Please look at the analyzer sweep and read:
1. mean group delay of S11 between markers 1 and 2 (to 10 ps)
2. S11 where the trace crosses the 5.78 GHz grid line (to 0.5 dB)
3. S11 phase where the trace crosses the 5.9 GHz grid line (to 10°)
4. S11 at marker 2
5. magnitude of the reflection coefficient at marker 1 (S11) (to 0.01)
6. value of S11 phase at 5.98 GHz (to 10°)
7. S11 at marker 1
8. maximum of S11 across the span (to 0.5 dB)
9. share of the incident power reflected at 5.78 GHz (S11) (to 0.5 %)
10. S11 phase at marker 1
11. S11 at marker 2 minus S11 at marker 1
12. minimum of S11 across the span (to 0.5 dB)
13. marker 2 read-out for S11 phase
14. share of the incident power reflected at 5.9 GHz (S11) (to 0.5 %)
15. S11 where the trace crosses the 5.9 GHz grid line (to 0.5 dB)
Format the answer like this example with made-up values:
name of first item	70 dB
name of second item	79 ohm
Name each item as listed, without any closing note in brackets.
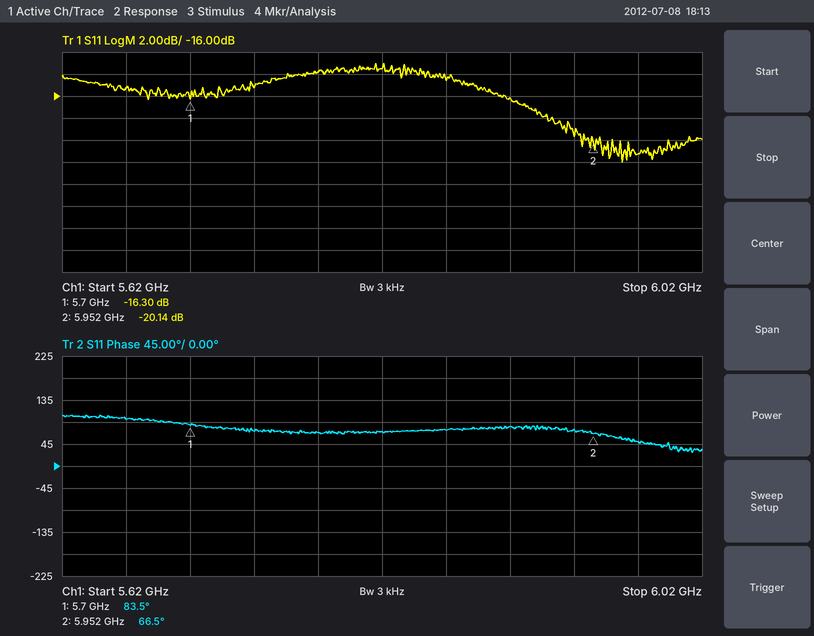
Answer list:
mean group delay of S11 between markers 1 and 2	190 ps
S11 where the trace crosses the 5.78 GHz grid line	-14.0 dB
S11 phase where the trace crosses the 5.9 GHz grid line	80°
S11 at marker 2	-20.14 dB
magnitude of the reflection coefficient at marker 1 (S11)	0.15
value of S11 phase at 5.98 GHz	50°
S11 at marker 1	-16.30 dB
maximum of S11 across the span	-13.0 dB
share of the incident power reflected at 5.78 GHz (S11)	4.0 %
S11 phase at marker 1	83.5°
S11 at marker 2 minus S11 at marker 1	-3.84 dB
minimum of S11 across the span	-22.0 dB
marker 2 read-out for S11 phase	66.5°
share of the incident power reflected at 5.9 GHz (S11)	2.5 %
S11 where the trace crosses the 5.9 GHz grid line	-16.0 dB
